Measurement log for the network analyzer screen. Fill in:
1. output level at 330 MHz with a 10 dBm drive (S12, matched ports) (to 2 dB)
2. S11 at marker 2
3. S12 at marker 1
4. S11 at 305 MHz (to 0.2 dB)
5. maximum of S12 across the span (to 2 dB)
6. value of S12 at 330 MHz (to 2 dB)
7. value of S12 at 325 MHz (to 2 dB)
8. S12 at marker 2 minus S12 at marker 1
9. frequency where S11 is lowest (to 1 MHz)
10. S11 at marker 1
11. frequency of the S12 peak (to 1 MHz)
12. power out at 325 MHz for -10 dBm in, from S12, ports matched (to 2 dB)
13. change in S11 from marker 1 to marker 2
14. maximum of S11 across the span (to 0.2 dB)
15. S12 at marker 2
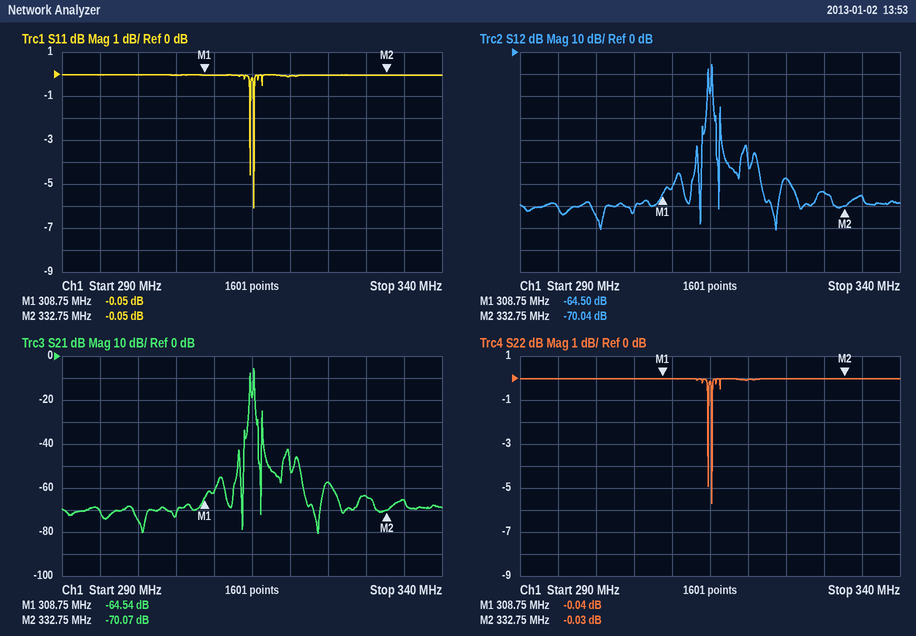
-54 dBm
-0.05 dB
-64.50 dB
0.0 dB
-6 dB
-64 dB
-58 dB
-5.54 dB
315 MHz
-0.05 dB
315 MHz
-68 dBm
0.00 dB
0.0 dB
-70.04 dB
